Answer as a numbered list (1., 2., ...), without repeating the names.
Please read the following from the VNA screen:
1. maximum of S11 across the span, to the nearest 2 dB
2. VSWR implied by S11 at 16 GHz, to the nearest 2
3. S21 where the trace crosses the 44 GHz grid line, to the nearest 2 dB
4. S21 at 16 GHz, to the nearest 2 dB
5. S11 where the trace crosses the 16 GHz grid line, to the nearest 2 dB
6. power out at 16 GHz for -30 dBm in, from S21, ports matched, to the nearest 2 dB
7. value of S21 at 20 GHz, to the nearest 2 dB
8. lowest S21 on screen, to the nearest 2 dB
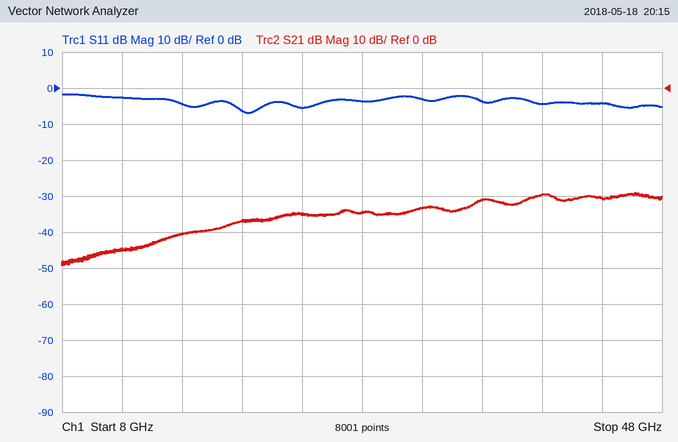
1. -2 dB
2. 4
3. -30 dB
4. -40 dB
5. -4 dB
6. -70 dBm
7. -36 dB
8. -50 dB
